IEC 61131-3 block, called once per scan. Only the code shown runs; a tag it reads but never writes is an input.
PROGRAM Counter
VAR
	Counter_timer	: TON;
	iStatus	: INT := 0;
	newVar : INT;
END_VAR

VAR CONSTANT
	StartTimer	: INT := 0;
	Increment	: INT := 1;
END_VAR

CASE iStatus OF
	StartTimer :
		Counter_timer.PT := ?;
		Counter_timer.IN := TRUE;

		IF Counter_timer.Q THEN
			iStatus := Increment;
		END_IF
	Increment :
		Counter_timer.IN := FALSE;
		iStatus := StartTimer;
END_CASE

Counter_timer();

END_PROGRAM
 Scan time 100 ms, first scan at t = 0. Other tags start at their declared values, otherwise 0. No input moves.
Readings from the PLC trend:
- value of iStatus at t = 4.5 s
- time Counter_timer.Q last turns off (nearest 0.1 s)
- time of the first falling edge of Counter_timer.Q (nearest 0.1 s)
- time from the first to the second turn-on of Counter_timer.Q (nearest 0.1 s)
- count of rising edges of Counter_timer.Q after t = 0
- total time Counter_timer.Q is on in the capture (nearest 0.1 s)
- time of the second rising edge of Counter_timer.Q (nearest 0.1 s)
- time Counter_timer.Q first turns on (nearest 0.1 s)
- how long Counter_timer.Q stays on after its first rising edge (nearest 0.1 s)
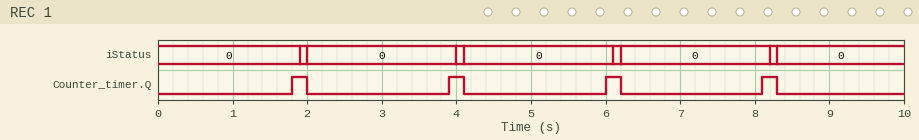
0
8.3 s
2.0 s
2.1 s
4
0.8 s
3.9 s
1.8 s
0.2 s
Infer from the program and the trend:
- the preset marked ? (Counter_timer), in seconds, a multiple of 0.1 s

1.8 s
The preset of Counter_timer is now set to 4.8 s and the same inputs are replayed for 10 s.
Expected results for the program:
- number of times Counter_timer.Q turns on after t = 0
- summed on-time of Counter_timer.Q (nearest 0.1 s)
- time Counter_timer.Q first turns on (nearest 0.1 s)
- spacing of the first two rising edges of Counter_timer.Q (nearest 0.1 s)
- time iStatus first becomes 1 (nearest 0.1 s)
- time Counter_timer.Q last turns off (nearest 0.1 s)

2
0.3 s
4.8 s
5.1 s
4.9 s
5.0 s
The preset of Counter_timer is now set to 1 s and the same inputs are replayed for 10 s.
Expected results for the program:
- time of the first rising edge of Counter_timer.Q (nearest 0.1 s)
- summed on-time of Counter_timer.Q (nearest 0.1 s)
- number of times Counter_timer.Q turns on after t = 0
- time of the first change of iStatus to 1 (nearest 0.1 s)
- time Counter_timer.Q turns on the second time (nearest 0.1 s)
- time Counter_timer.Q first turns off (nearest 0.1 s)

1.0 s
1.4 s
7
1.1 s
2.3 s
1.2 s
